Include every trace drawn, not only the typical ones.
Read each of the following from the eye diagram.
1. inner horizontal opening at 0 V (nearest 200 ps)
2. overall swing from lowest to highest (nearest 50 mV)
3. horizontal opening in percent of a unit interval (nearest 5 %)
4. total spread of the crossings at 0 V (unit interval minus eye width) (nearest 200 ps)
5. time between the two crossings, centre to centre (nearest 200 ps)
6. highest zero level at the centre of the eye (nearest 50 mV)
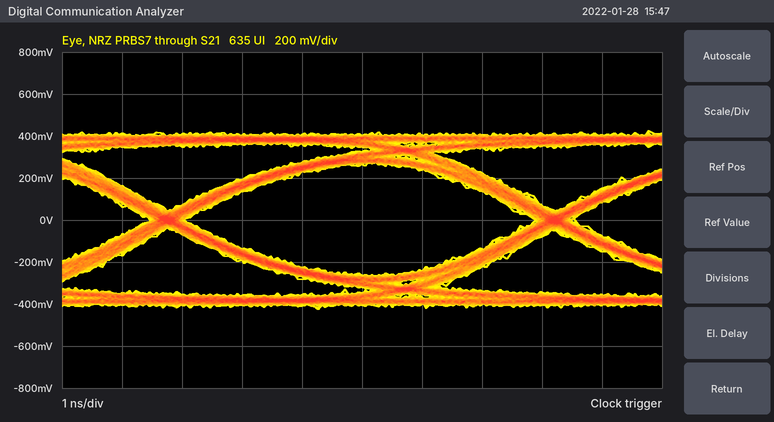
5.8 ns
850 mV
90 %
600 ps
6.4 ns
-250 mV
